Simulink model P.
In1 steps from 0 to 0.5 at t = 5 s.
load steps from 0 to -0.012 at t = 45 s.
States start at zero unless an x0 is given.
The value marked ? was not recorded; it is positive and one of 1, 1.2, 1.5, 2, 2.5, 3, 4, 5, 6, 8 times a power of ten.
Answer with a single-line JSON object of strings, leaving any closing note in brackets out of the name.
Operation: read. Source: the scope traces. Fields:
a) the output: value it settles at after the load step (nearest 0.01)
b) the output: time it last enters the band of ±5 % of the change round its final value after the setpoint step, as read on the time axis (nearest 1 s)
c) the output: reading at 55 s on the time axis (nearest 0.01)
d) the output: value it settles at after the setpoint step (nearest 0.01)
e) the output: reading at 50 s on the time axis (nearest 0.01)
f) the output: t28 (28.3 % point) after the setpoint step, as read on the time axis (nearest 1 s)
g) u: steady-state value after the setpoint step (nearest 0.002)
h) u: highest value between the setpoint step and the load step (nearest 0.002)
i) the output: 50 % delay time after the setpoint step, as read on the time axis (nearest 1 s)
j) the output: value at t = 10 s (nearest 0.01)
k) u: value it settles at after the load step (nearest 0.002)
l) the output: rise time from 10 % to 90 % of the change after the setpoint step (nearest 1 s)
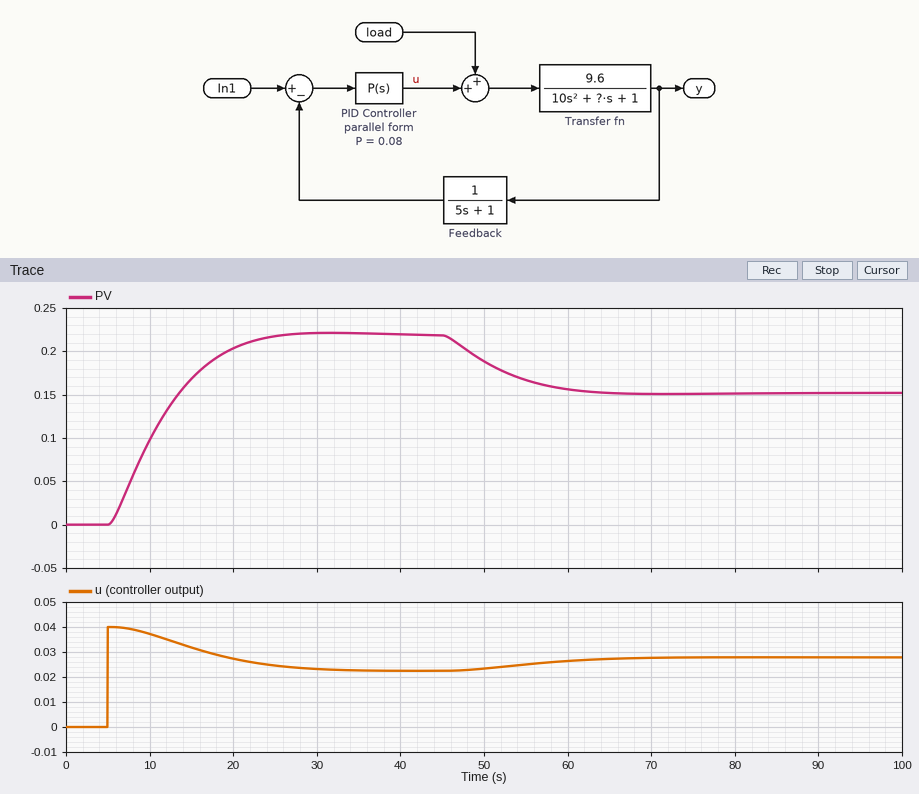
{"the output: value it settles at after the load step": "0.15", "the output: time it last enters the band of ±5 % of the change round its final value after the setpoint step, as read on the time axis": "21 s", "the output: reading at 55 s on the time axis": "0.17", "the output: value it settles at after the setpoint step": "0.22", "the output: reading at 50 s on the time axis": "0.19", "the output: t28 (28.3 % point) after the setpoint step, as read on the time axis": "8 s", "u: steady-state value after the setpoint step": "0.022", "u: highest value between the setpoint step and the load step": "0.040", "the output: 50 % delay time after the setpoint step, as read on the time axis": "11 s", "the output: value at t = 10 s": "0.10", "u: value it settles at after the load step": "0.028", "the output: rise time from 10 % to 90 % of the change after the setpoint step": "12 s"}
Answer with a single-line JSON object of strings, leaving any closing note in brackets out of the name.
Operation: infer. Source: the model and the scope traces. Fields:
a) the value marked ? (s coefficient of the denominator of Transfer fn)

{"the value marked ?": "15"}
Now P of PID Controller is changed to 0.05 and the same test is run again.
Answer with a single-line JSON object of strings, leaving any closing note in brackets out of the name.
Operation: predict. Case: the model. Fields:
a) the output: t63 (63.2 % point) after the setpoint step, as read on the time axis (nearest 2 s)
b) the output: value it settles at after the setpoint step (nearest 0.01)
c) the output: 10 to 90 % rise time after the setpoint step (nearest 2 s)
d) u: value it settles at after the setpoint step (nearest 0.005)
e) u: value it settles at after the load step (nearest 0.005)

{"the output: t63 (63.2 % point) after the setpoint step, as read on the time axis": "14 s", "the output: value it settles at after the setpoint step": "0.16", "the output: 10 to 90 % rise time after the setpoint step": "16 s", "u: value it settles at after the setpoint step": "0.015", "u: value it settles at after the load step": "0.020"}
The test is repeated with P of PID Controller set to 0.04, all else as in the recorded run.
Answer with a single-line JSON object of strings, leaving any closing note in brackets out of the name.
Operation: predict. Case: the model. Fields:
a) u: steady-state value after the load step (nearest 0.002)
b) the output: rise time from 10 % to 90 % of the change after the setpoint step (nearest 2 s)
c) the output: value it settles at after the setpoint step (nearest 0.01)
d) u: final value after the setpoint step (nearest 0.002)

{"u: steady-state value after the load step": "0.018", "the output: rise time from 10 % to 90 % of the change after the setpoint step": "18 s", "the output: value it settles at after the setpoint step": "0.14", "u: final value after the setpoint step": "0.014"}
